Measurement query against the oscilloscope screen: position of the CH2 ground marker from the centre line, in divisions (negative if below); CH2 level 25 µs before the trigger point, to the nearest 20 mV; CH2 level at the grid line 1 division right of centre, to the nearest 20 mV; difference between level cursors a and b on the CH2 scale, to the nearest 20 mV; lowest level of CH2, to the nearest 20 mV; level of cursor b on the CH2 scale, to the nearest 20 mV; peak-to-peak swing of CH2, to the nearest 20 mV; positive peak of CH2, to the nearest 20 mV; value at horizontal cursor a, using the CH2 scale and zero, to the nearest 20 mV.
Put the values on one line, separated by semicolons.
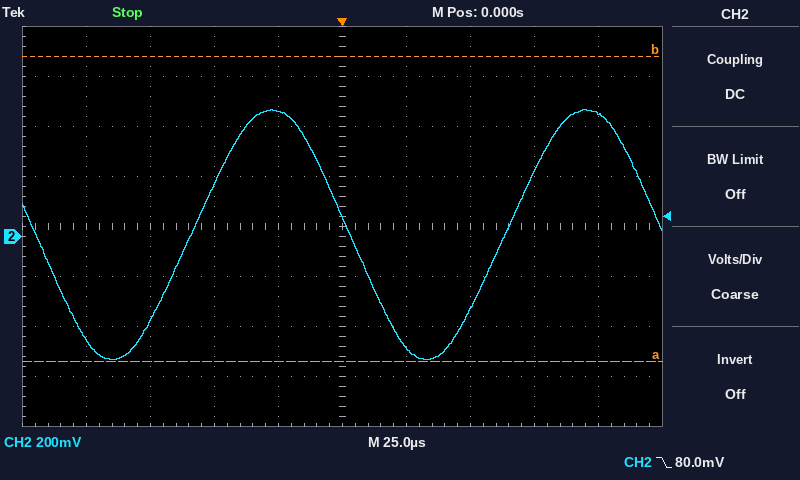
-0.2 div; 500 mV; -440 mV; 1.22 V; -500 mV; 720 mV; 1.00 V; 500 mV; -500 mV
